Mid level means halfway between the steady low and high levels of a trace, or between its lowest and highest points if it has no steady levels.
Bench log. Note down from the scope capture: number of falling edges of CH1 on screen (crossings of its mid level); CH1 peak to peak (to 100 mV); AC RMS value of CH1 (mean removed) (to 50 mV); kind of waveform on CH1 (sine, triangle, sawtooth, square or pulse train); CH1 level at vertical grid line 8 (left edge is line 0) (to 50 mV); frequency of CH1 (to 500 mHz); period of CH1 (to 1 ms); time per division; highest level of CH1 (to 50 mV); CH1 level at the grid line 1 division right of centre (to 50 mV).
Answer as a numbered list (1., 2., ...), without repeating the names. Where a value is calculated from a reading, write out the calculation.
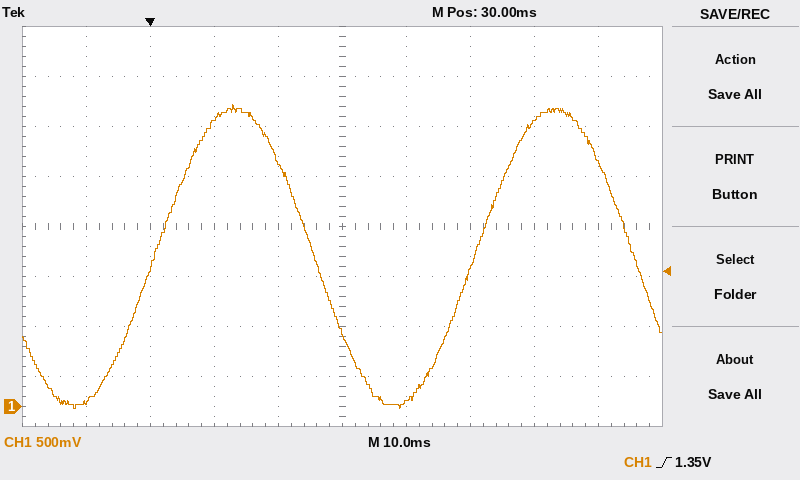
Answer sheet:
1. 2
2. 3.00 V
3. 3.00 V / (2√2) ≈ 1.06 V, so 1.05 V to the nearest 50 mV
4. sine
5. 2.85 V
6. 1 / 50 ms ≈ 20.0 Hz
7. 50 ms
8. 10 ms
9. 3.00 V
10. 50 mV
